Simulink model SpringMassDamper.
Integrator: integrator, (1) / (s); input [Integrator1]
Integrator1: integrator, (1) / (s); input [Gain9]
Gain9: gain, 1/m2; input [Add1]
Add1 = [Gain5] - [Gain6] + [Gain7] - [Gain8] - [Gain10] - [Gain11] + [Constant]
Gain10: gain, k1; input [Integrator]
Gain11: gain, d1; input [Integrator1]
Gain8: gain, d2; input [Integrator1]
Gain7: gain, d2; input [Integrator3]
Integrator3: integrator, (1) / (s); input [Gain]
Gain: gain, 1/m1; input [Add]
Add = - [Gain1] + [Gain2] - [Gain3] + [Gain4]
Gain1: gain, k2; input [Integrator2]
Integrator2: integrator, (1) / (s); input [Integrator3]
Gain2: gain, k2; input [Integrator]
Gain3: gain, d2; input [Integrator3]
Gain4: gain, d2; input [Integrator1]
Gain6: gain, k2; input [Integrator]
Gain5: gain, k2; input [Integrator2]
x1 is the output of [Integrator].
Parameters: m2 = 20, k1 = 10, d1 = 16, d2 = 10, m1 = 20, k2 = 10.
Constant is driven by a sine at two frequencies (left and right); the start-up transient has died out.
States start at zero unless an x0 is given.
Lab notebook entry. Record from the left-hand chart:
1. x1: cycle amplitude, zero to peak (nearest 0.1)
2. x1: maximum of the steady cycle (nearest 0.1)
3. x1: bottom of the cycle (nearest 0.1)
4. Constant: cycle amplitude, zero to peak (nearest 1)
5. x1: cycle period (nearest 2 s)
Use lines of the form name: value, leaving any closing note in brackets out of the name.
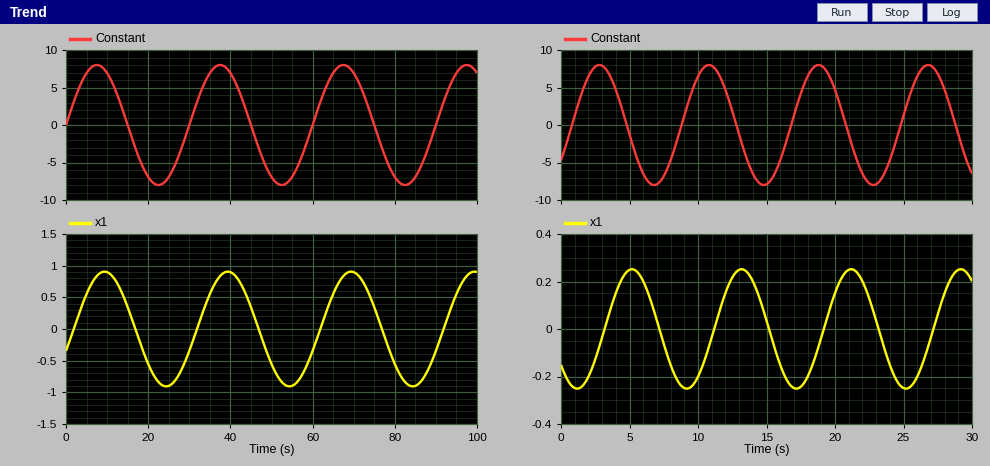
x1: cycle amplitude, zero to peak: 0.9
x1: maximum of the steady cycle: 0.9
x1: bottom of the cycle: -0.9
Constant: cycle amplitude, zero to peak: 8
x1: cycle period: 30 s
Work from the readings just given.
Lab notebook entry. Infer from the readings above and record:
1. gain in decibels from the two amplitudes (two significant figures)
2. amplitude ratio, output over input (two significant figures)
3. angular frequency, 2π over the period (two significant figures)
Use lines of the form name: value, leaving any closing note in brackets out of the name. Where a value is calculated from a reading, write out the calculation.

gain in decibels from the two amplitudes: 20 log10(0.9 / 8) = -19 dB
amplitude ratio, output over input: 0.9 / 8 = 0.11
angular frequency, 2π over the period: 2π / 30 = 0.21 rad/s
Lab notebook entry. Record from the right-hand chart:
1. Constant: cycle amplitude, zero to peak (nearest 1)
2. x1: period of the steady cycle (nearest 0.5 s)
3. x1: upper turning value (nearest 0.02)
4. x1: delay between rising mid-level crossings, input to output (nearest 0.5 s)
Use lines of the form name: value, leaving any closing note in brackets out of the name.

Constant: cycle amplitude, zero to peak: 8
x1: period of the steady cycle: 8.0 s
x1: upper turning value: 0.26
x1: delay between rising mid-level crossings, input to output: 2.5 s
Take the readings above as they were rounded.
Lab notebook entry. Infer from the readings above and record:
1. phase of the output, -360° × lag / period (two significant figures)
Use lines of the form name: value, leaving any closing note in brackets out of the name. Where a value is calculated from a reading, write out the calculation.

phase of the output, -360° × lag / period: -360 × 2.5 / 8 = -110°
